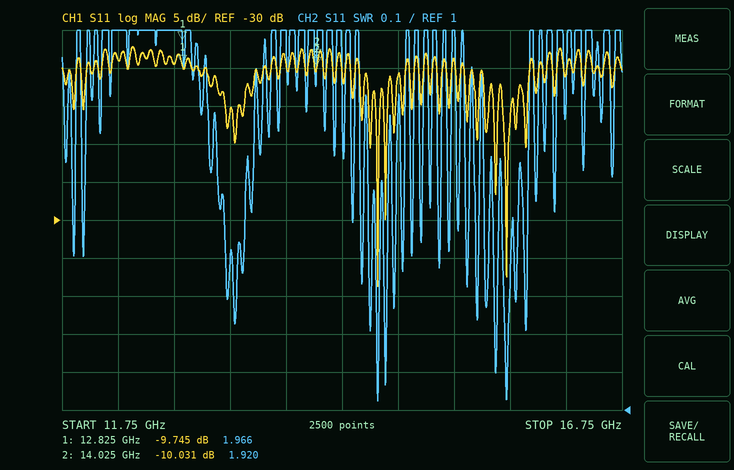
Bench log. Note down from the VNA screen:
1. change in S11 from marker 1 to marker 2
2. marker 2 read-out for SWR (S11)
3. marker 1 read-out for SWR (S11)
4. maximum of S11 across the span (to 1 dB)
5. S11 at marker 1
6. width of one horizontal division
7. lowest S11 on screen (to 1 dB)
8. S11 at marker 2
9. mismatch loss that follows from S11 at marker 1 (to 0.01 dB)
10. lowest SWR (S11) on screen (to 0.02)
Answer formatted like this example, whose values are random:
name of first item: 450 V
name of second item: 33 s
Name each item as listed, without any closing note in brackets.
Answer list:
change in S11 from marker 1 to marker 2: -0.286 dB
marker 2 read-out for SWR: 1.920
marker 1 read-out for SWR: 1.966
maximum of S11 across the span: -7 dB
S11 at marker 1: -9.745 dB
width of one horizontal division: 500 MHz
lowest S11 on screen: -39 dB
S11 at marker 2: -10.031 dB
mismatch loss that follows from S11 at marker 1: 0.49 dB
lowest SWR (S11) on screen: 1.02
